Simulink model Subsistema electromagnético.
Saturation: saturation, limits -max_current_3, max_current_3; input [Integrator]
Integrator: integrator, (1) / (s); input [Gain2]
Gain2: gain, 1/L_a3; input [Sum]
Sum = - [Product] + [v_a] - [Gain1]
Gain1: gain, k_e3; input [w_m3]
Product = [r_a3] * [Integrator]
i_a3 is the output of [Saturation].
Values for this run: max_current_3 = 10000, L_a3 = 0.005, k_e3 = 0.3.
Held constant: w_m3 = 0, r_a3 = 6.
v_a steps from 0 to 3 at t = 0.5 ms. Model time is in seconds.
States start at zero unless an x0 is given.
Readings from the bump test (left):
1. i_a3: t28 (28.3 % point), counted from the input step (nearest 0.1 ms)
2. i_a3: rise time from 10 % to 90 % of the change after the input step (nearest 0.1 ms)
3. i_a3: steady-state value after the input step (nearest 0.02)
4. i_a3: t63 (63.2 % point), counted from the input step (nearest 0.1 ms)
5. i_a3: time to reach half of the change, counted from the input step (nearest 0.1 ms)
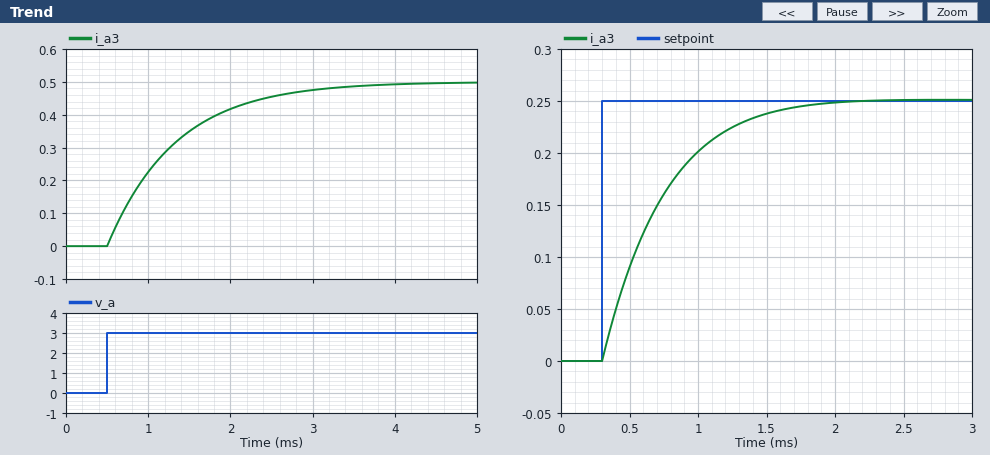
0.3 ms
1.8 ms
0.50
0.8 ms
0.6 ms
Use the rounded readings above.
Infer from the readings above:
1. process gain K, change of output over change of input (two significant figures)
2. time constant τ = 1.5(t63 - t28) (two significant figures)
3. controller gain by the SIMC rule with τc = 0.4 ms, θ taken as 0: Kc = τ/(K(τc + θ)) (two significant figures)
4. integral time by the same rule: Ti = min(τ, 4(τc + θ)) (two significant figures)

0.17
0.75 ms
11
0.75 ms
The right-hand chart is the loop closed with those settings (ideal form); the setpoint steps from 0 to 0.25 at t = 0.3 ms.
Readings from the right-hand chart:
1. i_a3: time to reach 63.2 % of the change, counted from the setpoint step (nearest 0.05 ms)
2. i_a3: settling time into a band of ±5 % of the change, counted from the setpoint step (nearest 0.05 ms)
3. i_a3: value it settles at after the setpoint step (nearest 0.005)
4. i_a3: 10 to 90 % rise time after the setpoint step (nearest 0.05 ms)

0.45 ms
1.20 ms
0.250
0.90 ms
